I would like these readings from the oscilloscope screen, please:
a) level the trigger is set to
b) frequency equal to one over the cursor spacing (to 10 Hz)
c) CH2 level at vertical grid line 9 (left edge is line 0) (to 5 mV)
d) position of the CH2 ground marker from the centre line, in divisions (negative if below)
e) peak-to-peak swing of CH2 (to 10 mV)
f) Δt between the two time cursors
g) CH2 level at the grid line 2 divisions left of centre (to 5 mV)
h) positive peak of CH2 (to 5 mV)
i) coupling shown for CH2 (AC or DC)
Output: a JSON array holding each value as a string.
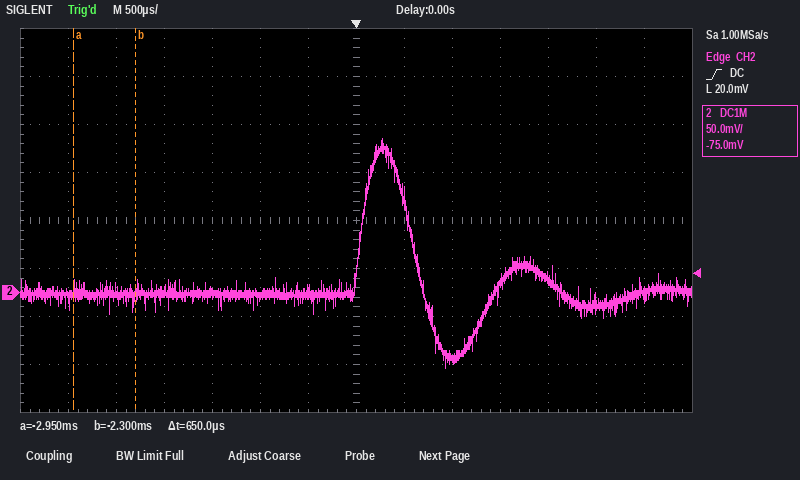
["20.0 mV", "1.54 kHz", "-70 mV", "-1.5 div", "240 mV", "650 µs", "-5 mV", "160 mV", "DC"]
